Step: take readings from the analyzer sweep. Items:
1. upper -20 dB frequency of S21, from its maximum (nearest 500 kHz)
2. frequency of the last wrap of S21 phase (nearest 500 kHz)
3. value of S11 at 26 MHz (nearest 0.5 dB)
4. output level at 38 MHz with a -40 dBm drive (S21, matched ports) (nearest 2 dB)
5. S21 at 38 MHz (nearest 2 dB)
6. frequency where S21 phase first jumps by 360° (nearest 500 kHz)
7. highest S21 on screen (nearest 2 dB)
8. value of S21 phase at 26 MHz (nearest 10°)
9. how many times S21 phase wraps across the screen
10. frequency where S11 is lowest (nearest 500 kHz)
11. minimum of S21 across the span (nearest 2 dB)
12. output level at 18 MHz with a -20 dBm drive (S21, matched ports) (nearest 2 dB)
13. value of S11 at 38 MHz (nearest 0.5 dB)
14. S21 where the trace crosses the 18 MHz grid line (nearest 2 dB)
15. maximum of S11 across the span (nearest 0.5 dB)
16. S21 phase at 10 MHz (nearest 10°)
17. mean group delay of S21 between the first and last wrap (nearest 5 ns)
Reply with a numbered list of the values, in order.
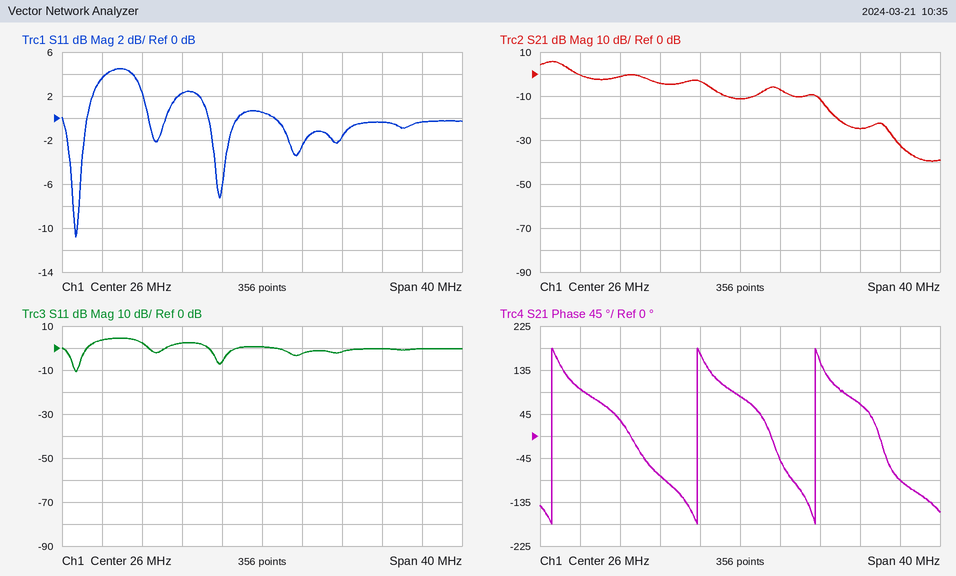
1. 34.5 MHz
2. 33.5 MHz
3. 0.5 dB
4. -64 dBm
5. -24 dB
6. 7.0 MHz
7. 6 dB
8. 80°
9. 3
10. 7.5 MHz
11. -40 dB
12. -24 dBm
13. -0.5 dB
14. -4 dB
15. 4.5 dB
16. 100°
17. 75 ns
